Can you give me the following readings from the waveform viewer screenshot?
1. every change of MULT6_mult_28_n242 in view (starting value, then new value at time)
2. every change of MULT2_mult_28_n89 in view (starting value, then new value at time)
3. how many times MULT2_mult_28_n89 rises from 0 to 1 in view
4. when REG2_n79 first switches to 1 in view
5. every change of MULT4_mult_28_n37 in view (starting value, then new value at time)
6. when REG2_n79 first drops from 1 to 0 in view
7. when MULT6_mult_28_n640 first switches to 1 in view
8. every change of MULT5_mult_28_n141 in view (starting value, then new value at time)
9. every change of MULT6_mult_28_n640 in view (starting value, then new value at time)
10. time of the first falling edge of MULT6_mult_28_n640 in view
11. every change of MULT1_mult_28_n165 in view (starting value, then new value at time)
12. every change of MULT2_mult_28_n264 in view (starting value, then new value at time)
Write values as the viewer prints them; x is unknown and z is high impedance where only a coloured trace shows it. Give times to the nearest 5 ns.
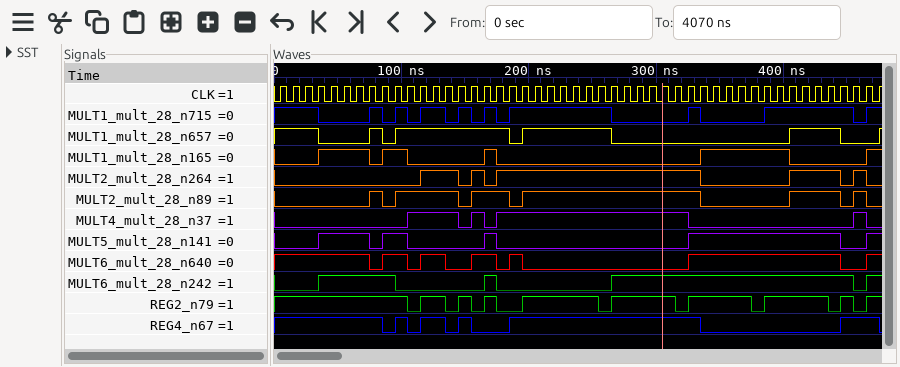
0, 1 at 35 ns, 0 at 95 ns, 1 at 165 ns, 0 at 175 ns, 1 at 265 ns, 0 at 455 ns, 1 at 465 ns
0, 1 at 75 ns, 0 at 85 ns, 1 at 95 ns, 0 at 145 ns, 1 at 155 ns, 0 at 185 ns, 1 at 195 ns, 0 at 335 ns, 1 at 405 ns, 0 at 445 ns, 1 at 455 ns, 0 at 465 ns
6
115 ns
0, 1 at 105 ns, 0 at 145 ns, 1 at 155 ns, 0 at 165 ns, 1 at 175 ns, 0 at 325 ns, 1 at 455 ns, 0 at 465 ns
105 ns
85 ns
0, 1 at 35 ns, 0 at 75 ns, 1 at 85 ns, 0 at 105 ns, 1 at 165 ns, 0 at 175 ns, 1 at 325 ns, 0 at 445 ns, 1 at 465 ns
1, 0 at 75 ns, 1 at 85 ns, 0 at 105 ns, 1 at 115 ns, 0 at 135 ns, 1 at 155 ns, 0 at 175 ns, 1 at 185 ns, 0 at 195 ns, 1 at 325 ns, 0 at 445 ns, 1 at 465 ns
75 ns
0, 1 at 35 ns, 0 at 75 ns, 1 at 85 ns, 0 at 105 ns, 1 at 165 ns, 0 at 175 ns, 1 at 335 ns, 0 at 405 ns, 1 at 465 ns
0, 1 at 115 ns, 0 at 145 ns, 1 at 155 ns, 0 at 165 ns, 1 at 175 ns, 0 at 335 ns, 1 at 405 ns, 0 at 445 ns, 1 at 455 ns, 0 at 465 ns
